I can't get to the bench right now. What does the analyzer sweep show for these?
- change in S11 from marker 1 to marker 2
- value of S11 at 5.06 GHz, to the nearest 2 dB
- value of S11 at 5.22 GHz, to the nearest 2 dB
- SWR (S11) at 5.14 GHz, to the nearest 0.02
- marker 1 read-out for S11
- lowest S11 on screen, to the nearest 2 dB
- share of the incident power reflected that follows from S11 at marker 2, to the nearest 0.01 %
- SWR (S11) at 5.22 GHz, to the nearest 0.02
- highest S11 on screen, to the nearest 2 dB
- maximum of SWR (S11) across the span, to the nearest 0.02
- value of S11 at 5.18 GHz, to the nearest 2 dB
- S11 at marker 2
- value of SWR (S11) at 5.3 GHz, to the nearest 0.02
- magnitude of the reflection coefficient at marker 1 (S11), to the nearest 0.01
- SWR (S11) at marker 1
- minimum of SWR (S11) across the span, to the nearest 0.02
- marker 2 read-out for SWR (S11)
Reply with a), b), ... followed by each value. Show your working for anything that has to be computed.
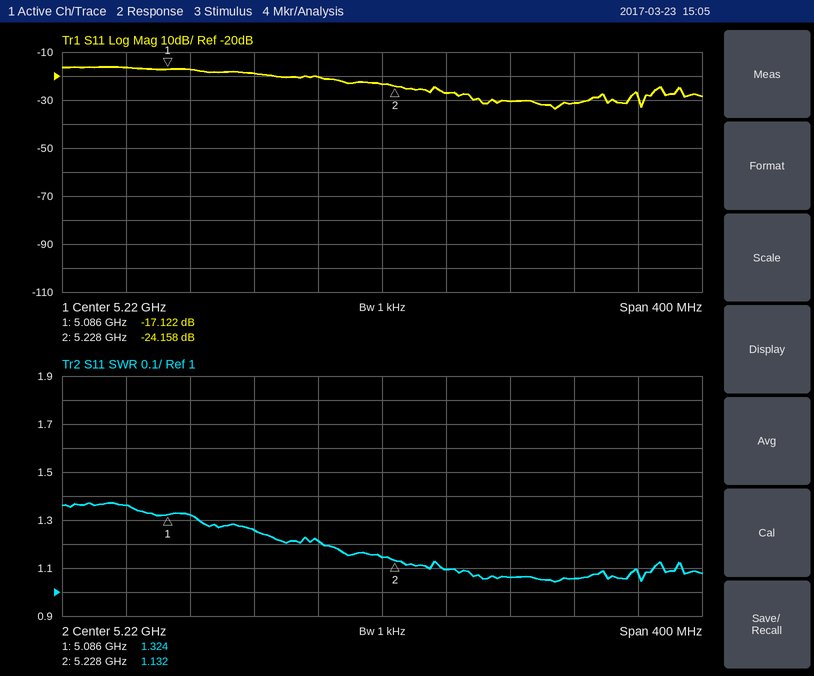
a) -24.158 − (-17.122) = -7.036 dB
b) -16 dB
c) -24 dB
d) 1.26
e) -17.122 dB
f) -34 dB
g) 10^(-24.158/10) ≈ 0.38 %
h) 1.14
i) -16 dB
j) 1.38
k) -20 dB
l) -24.158 dB
m) 1.06
n) 10^(-17.122/20) ≈ 0.14
o) 1.324
p) 1.04
q) 1.132
